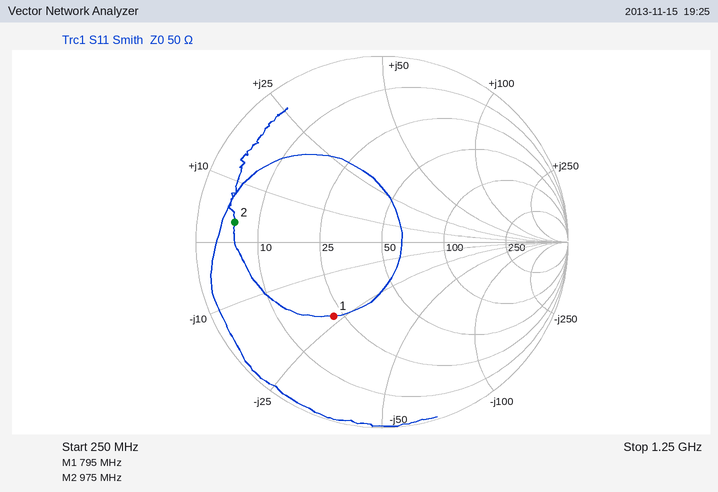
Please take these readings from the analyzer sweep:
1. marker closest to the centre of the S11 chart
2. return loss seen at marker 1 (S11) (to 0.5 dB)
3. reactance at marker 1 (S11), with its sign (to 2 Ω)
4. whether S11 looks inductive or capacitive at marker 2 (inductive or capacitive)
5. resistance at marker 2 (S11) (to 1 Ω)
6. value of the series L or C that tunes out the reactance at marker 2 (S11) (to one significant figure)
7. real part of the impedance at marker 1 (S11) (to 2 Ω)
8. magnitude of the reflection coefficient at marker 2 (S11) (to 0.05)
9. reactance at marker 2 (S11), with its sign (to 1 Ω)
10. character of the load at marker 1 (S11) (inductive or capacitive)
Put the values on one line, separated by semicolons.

marker 1; 6.5 dB; -22 Ω; inductive; 6 Ω; 50 pF; 22 Ω; 0.80; +3 Ω; capacitive
